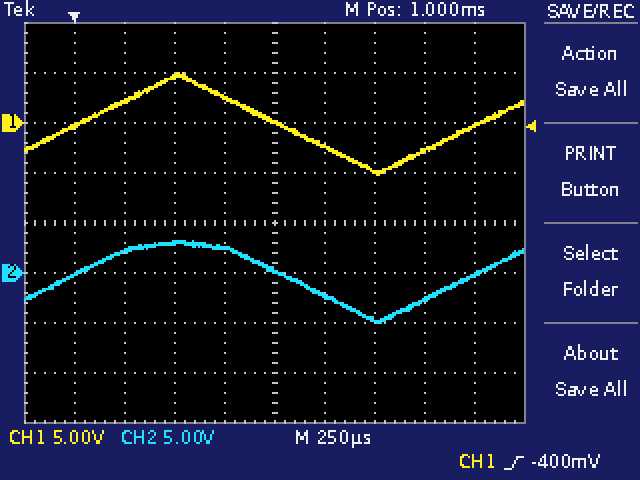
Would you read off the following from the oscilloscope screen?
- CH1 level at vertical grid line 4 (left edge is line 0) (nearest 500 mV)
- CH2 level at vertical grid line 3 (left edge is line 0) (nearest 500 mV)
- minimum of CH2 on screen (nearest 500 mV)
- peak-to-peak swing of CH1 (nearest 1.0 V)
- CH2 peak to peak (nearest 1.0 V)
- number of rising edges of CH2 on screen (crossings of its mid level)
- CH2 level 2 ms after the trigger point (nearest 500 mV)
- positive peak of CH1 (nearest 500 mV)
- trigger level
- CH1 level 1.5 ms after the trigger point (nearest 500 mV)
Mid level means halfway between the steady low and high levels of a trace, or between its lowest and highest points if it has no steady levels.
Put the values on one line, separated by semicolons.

2.5 V; 3.0 V; -5.0 V; 10.0 V; 8.0 V; 2; 0.0 V; 5.0 V; -400 mV; -5.0 V
